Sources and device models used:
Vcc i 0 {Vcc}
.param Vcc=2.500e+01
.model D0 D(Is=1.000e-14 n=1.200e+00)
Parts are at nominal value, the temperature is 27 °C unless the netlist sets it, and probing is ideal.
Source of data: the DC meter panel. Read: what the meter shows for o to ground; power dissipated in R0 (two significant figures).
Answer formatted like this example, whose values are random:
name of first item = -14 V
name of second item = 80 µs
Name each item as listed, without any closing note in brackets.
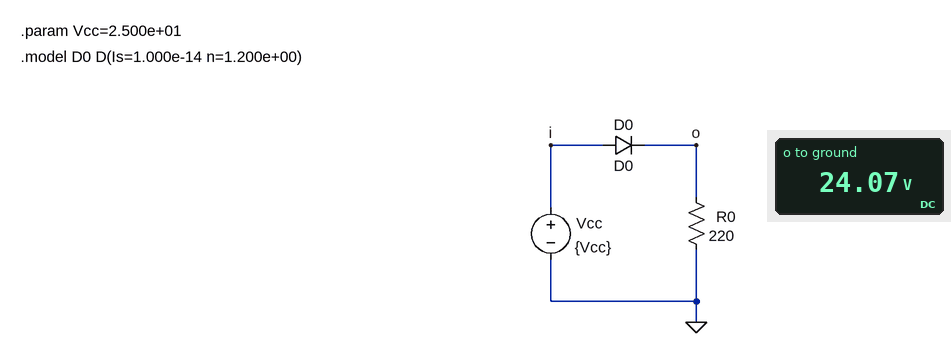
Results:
what the meter shows for o to ground = 24.07 V
power dissipated in R0 = 2.6 W
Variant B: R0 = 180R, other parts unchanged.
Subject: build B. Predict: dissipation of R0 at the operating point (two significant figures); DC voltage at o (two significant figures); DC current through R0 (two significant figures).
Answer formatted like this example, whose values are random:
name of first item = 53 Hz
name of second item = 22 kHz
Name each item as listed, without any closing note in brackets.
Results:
dissipation of R0 at the operating point = 3.2 W
DC voltage at o = 24 V
DC current through R0 = 130 mA
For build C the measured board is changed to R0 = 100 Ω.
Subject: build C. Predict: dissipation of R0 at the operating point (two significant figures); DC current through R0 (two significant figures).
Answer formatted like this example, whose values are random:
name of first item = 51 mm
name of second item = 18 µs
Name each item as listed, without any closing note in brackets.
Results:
dissipation of R0 at the operating point = 5.8 W
DC current through R0 = 240 mA
